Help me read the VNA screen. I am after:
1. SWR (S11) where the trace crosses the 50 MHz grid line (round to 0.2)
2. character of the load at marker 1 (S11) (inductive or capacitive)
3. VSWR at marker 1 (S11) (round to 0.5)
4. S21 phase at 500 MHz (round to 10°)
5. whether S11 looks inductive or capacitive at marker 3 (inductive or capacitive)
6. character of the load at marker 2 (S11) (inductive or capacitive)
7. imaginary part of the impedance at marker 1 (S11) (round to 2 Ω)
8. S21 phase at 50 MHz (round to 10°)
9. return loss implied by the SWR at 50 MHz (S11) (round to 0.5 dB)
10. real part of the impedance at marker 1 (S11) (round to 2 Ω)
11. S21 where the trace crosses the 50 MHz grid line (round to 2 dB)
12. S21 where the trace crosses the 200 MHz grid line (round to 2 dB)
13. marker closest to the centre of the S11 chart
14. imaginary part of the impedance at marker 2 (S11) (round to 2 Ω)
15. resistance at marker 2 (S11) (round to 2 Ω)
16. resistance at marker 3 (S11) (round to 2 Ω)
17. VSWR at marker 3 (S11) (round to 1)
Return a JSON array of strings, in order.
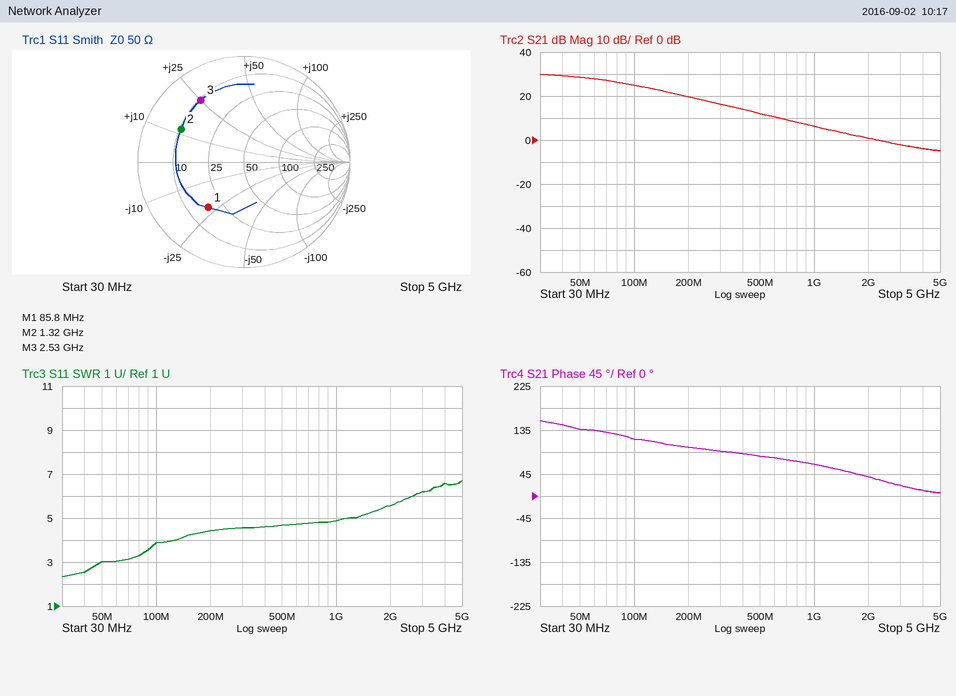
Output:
["3.0", "capacitive", "3.5", "80°", "inductive", "inductive", "-22 Ω", "140°", "6.0 dB", "18 Ω", "28 dB", "20 dB", "marker 1", "+12 Ω", "10 Ω", "10 Ω", "6"]
